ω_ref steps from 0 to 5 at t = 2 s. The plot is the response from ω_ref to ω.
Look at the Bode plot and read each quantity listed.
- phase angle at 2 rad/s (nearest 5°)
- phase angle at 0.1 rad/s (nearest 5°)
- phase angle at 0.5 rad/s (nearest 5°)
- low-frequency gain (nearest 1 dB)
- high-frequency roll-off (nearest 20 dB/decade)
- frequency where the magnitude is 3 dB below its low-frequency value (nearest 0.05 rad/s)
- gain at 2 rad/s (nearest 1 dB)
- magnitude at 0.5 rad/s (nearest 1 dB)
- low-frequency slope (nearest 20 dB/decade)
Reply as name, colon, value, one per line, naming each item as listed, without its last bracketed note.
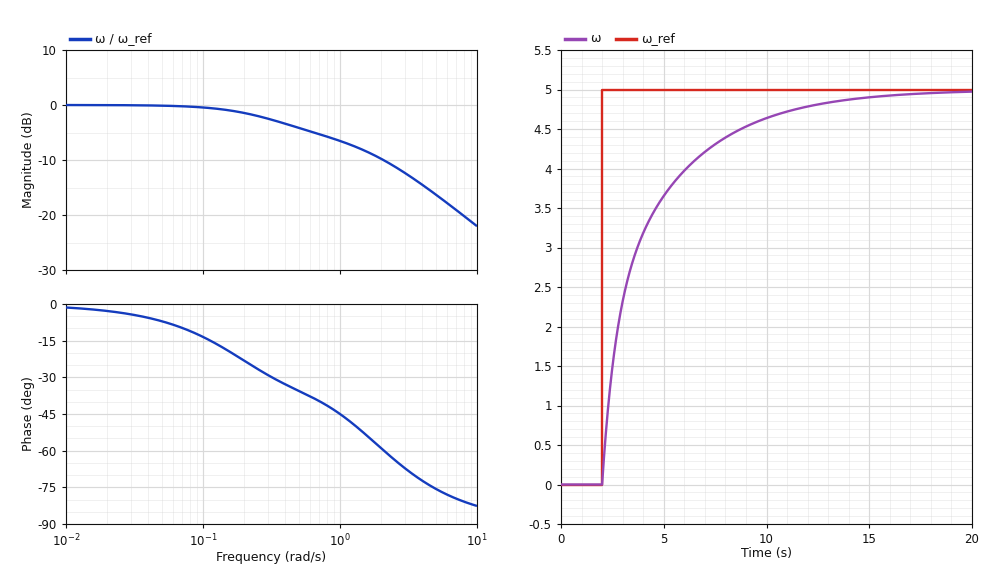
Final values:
phase angle at 2 rad/s: -60°
phase angle at 0.1 rad/s: -15°
phase angle at 0.5 rad/s: -35°
low-frequency gain: 0 dB
high-frequency roll-off: -20 dB/decade
frequency where the magnitude is 3 dB below its low-frequency value: 0.35 rad/s
gain at 2 rad/s: -10 dB
magnitude at 0.5 rad/s: -4 dB
low-frequency slope: 0 dB/decade
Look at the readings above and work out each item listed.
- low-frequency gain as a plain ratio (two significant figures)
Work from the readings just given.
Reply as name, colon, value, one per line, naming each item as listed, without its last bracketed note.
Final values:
low-frequency gain as a plain ratio: 1.0
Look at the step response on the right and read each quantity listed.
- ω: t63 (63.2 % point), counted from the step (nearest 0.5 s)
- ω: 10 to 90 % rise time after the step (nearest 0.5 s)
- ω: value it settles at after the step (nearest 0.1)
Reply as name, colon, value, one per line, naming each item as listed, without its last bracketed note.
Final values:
ω: t63 (63.2 % point), counted from the step: 2.0 s
ω: 10 to 90 % rise time after the step: 6.5 s
ω: value it settles at after the step: 5.0
